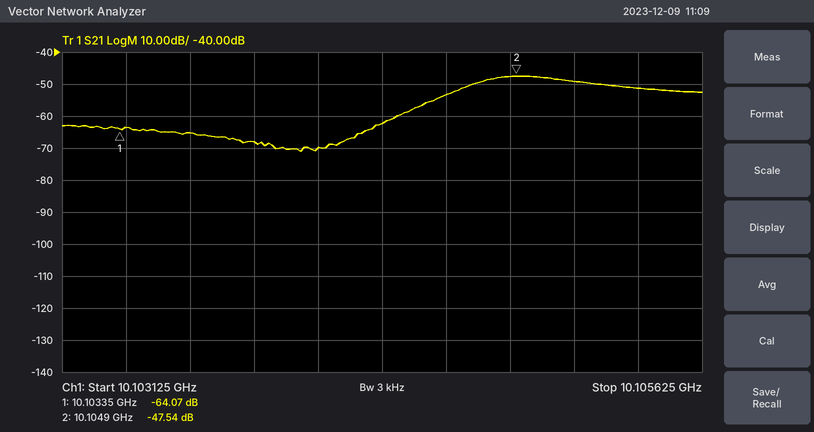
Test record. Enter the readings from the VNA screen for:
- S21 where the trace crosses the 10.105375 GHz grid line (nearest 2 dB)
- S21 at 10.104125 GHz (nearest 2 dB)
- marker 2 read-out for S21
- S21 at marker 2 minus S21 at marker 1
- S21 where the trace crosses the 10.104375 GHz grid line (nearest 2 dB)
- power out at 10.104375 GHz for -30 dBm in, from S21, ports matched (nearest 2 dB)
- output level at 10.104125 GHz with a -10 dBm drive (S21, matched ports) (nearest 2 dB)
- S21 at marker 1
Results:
-52 dB
-70 dB
-47.54 dB
16.53 dB
-62 dB
-92 dBm
-80 dBm
-64.07 dB
